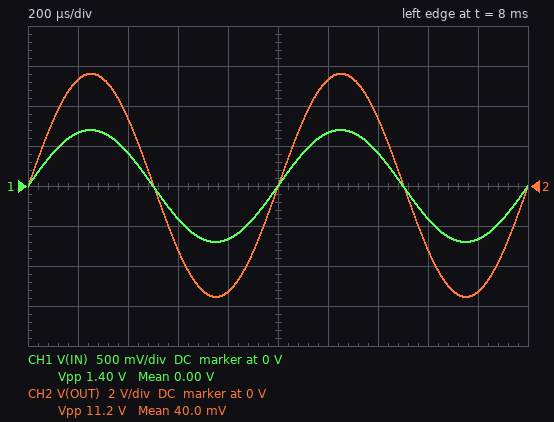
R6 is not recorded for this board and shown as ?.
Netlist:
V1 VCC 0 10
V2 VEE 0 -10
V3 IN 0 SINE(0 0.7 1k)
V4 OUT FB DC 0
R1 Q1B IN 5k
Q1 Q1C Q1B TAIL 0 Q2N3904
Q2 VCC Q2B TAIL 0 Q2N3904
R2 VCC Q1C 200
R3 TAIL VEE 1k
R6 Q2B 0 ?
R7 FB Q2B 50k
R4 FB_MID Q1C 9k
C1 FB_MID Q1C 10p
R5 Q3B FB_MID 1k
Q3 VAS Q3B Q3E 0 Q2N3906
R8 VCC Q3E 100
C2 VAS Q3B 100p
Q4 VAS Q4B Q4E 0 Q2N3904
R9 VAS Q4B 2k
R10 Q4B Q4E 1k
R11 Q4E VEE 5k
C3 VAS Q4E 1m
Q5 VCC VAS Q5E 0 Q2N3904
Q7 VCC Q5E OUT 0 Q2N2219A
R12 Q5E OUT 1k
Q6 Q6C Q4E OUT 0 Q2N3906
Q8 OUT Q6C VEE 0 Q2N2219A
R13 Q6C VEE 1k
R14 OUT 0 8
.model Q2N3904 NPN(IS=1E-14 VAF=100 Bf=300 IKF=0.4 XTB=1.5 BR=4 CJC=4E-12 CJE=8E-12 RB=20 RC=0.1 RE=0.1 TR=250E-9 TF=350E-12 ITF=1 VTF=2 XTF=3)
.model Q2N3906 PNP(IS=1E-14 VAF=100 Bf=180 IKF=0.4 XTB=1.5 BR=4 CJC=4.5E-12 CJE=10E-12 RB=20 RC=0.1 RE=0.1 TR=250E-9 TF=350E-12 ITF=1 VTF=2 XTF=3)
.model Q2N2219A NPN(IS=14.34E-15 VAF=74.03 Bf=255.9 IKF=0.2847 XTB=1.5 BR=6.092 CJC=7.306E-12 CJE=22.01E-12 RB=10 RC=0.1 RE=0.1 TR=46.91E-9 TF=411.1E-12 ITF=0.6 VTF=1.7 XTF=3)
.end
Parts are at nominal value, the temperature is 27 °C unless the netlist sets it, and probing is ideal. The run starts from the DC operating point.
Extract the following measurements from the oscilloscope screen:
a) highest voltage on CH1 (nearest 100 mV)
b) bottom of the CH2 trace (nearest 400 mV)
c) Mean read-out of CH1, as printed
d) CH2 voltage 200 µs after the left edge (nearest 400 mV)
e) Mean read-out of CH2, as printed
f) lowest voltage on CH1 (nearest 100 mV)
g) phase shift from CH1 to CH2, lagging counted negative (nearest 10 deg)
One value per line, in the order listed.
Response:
700 mV
-5.6 V
0.00 V
5.2 V
40.0 mV
-700 mV
0 deg
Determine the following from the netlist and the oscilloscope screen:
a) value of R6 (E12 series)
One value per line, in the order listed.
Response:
6.8 kΩ
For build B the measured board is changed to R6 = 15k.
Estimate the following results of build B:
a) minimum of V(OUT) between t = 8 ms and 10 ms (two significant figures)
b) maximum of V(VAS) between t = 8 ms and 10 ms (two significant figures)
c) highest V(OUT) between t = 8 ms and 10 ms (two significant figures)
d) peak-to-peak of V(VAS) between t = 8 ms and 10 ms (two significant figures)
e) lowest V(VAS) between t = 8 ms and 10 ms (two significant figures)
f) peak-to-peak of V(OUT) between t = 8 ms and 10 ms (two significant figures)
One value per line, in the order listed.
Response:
-2.7 V
4.9 V
3.3 V
6.3 V
-1.4 V
6.0 V
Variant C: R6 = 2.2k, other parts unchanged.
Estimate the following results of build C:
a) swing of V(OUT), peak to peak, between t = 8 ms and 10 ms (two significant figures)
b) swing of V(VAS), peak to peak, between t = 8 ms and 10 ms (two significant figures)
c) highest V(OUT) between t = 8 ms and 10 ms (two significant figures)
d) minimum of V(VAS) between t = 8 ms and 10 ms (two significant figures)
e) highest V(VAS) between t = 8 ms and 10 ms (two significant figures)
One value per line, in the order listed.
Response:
16 V
17 V
7.7 V
-7.4 V
9.6 V
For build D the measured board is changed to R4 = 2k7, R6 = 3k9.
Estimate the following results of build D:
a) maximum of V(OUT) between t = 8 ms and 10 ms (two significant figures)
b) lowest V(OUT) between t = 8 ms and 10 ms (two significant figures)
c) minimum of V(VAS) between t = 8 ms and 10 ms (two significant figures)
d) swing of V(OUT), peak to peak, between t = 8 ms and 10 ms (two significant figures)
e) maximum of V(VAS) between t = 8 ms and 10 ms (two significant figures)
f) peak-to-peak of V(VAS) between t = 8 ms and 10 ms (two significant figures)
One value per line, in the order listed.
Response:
7.7 V
-8.6 V
-7.4 V
16 V
9.6 V
17 V
